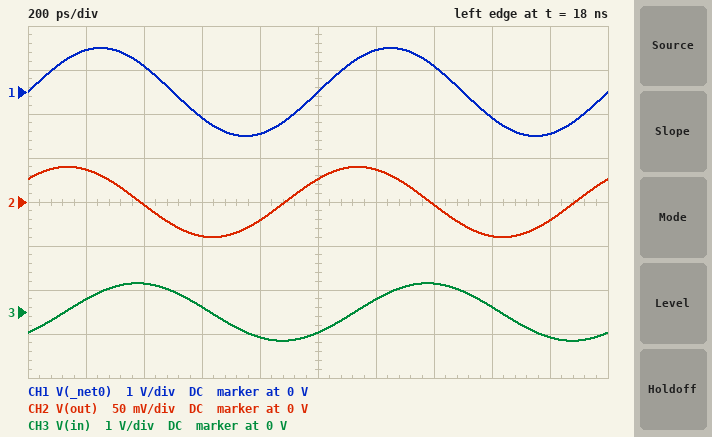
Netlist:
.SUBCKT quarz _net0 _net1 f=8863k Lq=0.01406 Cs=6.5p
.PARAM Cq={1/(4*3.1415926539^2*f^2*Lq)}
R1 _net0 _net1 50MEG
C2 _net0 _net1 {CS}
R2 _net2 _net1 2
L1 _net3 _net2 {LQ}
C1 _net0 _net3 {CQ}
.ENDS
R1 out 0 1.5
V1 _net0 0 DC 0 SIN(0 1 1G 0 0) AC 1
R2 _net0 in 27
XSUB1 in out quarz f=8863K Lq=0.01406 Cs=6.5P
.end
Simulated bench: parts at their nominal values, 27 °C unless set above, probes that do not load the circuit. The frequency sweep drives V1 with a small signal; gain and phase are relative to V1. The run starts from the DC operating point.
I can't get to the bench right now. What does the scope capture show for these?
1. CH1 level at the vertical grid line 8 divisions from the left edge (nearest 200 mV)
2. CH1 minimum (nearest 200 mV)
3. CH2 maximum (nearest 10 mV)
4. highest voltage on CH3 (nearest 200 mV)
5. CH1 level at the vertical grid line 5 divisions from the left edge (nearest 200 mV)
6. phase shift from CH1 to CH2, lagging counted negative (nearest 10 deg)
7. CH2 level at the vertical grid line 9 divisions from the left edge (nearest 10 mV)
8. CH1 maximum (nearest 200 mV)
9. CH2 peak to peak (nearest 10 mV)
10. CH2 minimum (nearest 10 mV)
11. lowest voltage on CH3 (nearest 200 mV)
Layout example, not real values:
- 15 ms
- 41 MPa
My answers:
- -600 mV
- -1.0 V
- 40 mV
- 600 mV
- 0 V
- 40 deg
- -20 mV
- 1.0 V
- 80 mV
- -40 mV
- -600 mV
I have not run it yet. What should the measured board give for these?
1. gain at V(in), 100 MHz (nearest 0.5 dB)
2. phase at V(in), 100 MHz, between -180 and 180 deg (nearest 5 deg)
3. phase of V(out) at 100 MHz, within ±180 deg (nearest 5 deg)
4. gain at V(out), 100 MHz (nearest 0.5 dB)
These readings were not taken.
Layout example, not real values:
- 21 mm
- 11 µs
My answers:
- 0 dB
- -5 deg
- 85 deg
- -44.5 dB
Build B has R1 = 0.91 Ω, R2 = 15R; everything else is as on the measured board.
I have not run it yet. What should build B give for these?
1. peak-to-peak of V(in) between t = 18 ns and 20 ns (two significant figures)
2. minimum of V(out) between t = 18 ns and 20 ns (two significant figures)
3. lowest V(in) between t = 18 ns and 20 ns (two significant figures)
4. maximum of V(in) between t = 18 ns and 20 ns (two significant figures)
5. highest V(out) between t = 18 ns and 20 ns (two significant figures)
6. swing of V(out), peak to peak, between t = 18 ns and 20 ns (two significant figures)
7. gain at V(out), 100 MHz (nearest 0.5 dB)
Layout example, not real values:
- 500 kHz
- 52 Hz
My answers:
- 1.7 V
- -31 mV
- -840 mV
- 840 mV
- 31 mV
- 62 mV
- -48.5 dB
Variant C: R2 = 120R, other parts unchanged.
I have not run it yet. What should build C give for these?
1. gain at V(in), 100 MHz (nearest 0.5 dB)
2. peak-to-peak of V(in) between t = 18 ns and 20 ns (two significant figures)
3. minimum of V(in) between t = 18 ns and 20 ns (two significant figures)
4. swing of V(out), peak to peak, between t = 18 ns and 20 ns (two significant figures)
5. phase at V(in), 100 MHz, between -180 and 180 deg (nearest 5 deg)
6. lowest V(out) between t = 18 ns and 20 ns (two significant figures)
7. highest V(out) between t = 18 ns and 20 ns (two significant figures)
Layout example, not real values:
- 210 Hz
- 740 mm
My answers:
- -1.0 dB
- 400 mV
- -200 mV
- 24 mV
- -25 deg
- -12 mV
- 12 mV
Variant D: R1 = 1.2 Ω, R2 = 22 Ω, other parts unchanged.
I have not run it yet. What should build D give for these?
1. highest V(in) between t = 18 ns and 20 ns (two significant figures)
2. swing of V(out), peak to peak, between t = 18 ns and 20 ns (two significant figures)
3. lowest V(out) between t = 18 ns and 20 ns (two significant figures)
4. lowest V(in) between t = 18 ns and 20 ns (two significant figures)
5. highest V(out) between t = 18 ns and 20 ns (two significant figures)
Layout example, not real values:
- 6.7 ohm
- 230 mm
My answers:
- 730 mV
- 71 mV
- -36 mV
- -730 mV
- 36 mV
